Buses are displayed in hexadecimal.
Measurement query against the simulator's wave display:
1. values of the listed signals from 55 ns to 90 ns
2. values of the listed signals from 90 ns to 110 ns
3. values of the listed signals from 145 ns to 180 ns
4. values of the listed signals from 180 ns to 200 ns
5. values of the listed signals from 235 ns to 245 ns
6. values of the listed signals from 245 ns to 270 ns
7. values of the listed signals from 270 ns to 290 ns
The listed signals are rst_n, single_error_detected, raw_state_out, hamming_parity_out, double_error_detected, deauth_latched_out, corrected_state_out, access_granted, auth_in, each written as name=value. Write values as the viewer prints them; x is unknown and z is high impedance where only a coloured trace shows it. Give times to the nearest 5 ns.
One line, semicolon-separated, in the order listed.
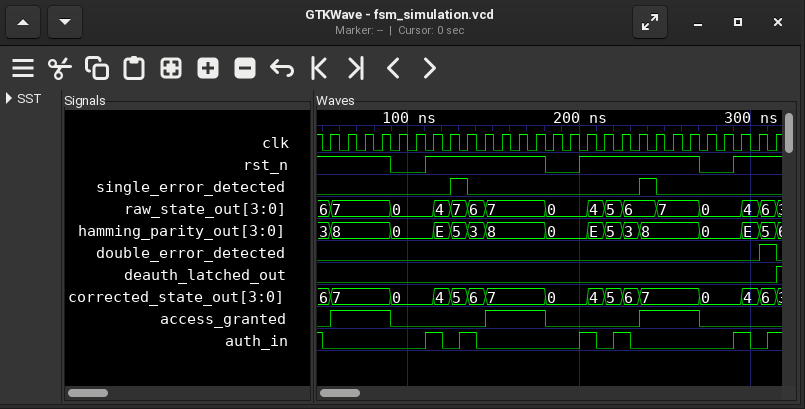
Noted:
rst_n=1, single_error_detected=0, raw_state_out=7, hamming_parity_out=8, double_error_detected=0, deauth_latched_out=0, corrected_state_out=7, access_granted=1, auth_in=0; rst_n=0, single_error_detected=0, raw_state_out=0, hamming_parity_out=0, double_error_detected=0, deauth_latched_out=0, corrected_state_out=0, access_granted=0, auth_in=0; rst_n=1, single_error_detected=0, raw_state_out=7, hamming_parity_out=8, double_error_detected=0, deauth_latched_out=0, corrected_state_out=7, access_granted=1, auth_in=0; rst_n=0, single_error_detected=0, raw_state_out=0, hamming_parity_out=0, double_error_detected=0, deauth_latched_out=0, corrected_state_out=0, access_granted=0, auth_in=0; rst_n=1, single_error_detected=1, raw_state_out=6, hamming_parity_out=8, double_error_detected=0, deauth_latched_out=0, corrected_state_out=7, access_granted=1, auth_in=0; rst_n=1, single_error_detected=0, raw_state_out=7, hamming_parity_out=8, double_error_detected=0, deauth_latched_out=0, corrected_state_out=7, access_granted=1, auth_in=0; rst_n=0, single_error_detected=0, raw_state_out=0, hamming_parity_out=0, double_error_detected=0, deauth_latched_out=0, corrected_state_out=0, access_granted=0, auth_in=0
